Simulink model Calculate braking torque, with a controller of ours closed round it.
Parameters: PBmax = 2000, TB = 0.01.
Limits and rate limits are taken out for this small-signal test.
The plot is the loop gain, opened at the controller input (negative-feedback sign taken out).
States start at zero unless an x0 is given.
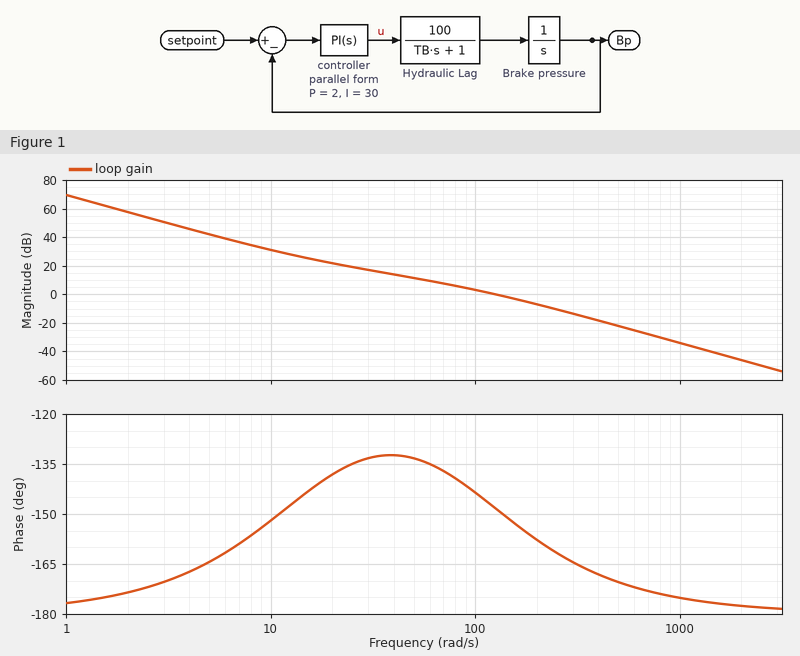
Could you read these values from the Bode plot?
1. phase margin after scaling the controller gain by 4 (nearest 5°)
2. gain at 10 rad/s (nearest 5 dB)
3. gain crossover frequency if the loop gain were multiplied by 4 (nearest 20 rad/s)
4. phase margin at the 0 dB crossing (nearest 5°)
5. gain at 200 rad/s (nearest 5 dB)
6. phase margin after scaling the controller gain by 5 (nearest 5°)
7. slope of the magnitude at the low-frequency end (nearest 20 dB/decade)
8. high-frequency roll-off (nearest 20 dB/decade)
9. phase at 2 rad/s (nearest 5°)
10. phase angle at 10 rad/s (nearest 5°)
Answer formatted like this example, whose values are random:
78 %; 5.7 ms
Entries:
15°; 30 dB; 280 rad/s; 30°; -5 dB; 15°; -40 dB/decade; -40 dB/decade; -175°; -150°
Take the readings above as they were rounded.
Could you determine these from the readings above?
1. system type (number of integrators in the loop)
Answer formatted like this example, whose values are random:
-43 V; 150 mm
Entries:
2
